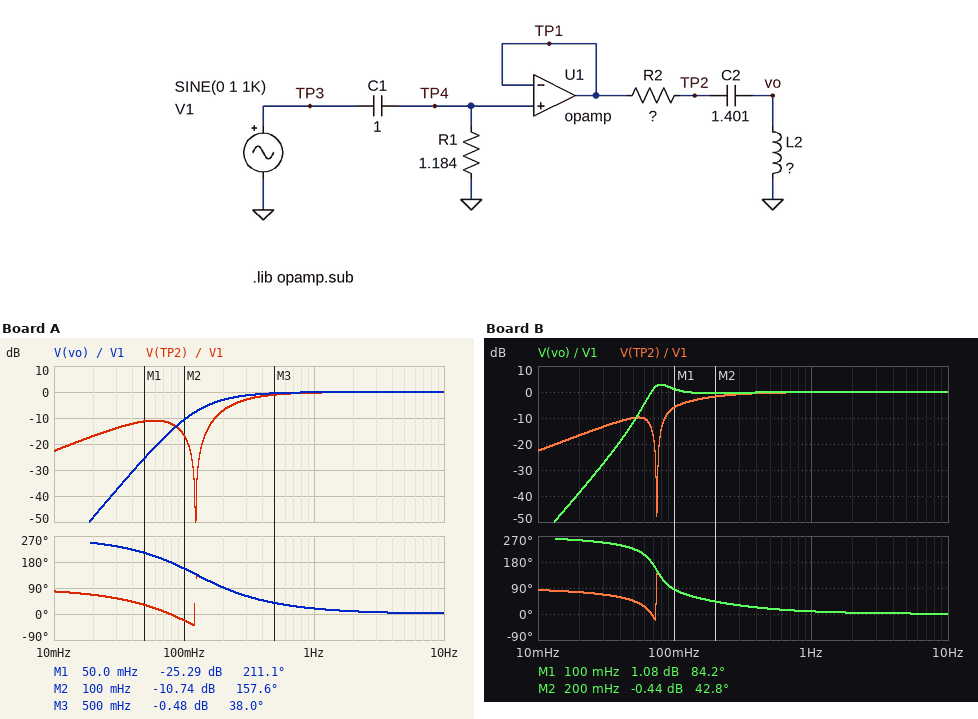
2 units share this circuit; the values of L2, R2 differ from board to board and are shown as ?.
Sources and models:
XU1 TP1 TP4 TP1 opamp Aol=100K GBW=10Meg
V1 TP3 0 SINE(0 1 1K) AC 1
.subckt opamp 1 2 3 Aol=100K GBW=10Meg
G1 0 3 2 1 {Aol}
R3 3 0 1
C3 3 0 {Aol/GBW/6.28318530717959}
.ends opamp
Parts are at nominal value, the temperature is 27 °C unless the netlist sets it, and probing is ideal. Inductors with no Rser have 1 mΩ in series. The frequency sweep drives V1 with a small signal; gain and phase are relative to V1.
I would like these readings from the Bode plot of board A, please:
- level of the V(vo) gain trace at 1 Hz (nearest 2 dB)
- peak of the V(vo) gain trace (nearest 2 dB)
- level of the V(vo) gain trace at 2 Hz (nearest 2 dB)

0 dB
0 dB
0 dB
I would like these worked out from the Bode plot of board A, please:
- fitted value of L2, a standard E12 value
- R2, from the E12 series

1.2 H
1.5 Ω
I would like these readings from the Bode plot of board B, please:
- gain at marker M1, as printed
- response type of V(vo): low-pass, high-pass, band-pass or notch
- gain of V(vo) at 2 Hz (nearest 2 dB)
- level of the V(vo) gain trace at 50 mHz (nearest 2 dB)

1.08 dB
high-pass
0 dB
-12 dB
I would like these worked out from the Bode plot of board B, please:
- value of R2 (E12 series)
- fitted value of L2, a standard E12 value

0.56 Ω
3.3 H
